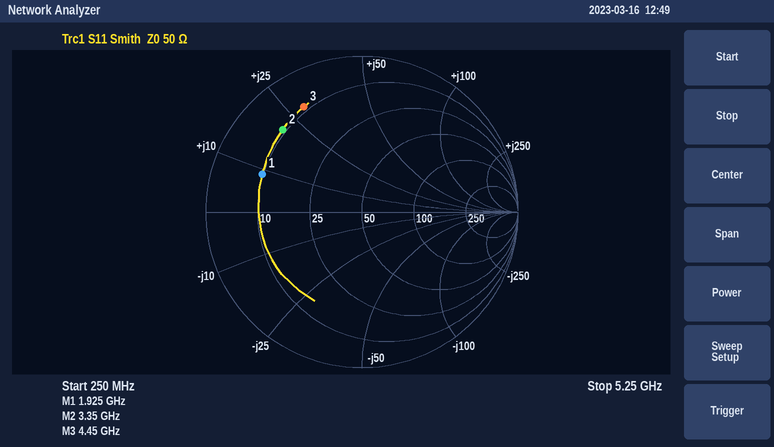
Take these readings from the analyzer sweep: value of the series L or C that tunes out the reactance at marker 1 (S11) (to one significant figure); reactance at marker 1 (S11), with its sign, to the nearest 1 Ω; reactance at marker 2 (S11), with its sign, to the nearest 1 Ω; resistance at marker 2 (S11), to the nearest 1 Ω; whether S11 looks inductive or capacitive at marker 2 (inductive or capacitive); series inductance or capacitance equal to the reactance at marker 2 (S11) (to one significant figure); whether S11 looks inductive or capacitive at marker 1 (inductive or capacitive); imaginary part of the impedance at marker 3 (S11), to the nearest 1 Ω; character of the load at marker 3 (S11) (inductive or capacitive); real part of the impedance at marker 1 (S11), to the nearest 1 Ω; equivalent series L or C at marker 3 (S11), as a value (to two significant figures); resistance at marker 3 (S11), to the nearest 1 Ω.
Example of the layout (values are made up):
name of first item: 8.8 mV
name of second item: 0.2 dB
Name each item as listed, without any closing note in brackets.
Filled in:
value of the series L or C that tunes out the reactance at marker 1 (S11): 9 pF
reactance at marker 1 (S11), with its sign, to the nearest 1 Ω: +9 Ω
reactance at marker 2 (S11), with its sign, to the nearest 1 Ω: +21 Ω
resistance at marker 2 (S11), to the nearest 1 Ω: 9 Ω
whether S11 looks inductive or capacitive at marker 2: inductive
series inductance or capacitance equal to the reactance at marker 2 (S11): 1.0 nH
whether S11 looks inductive or capacitive at marker 1: inductive
imaginary part of the impedance at marker 3 (S11), to the nearest 1 Ω: +29 Ω
character of the load at marker 3 (S11): inductive
real part of the impedance at marker 1 (S11), to the nearest 1 Ω: 10 Ω
equivalent series L or C at marker 3 (S11), as a value: 1.0 nH
resistance at marker 3 (S11), to the nearest 1 Ω: 9 Ω
